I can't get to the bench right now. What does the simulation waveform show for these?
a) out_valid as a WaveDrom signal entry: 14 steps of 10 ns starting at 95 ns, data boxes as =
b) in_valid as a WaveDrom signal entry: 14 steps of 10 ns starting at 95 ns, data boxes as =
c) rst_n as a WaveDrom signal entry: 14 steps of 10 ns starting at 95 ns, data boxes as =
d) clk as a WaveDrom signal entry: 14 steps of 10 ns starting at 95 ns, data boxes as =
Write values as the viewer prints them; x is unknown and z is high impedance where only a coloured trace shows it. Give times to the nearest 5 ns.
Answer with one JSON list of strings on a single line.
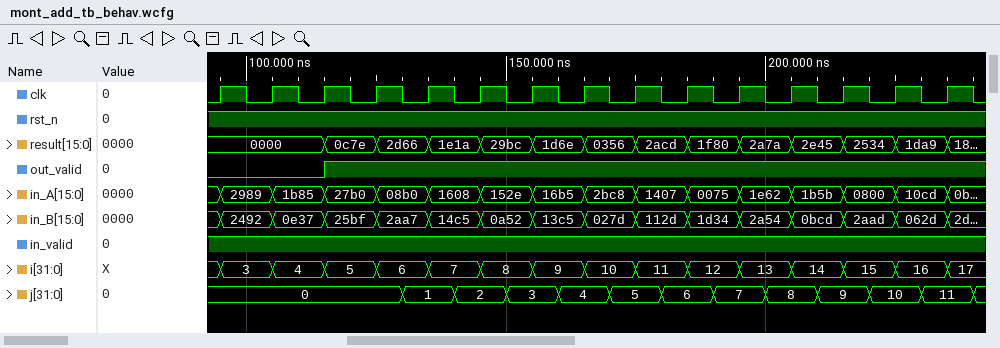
["{name: 'out_valid', wave: '0.1...........'}", "{name: 'in_valid', wave: '1.............'}", "{name: 'rst_n', wave: '1.............'}", "{name: 'clk', wave: 'p.............'}"]
